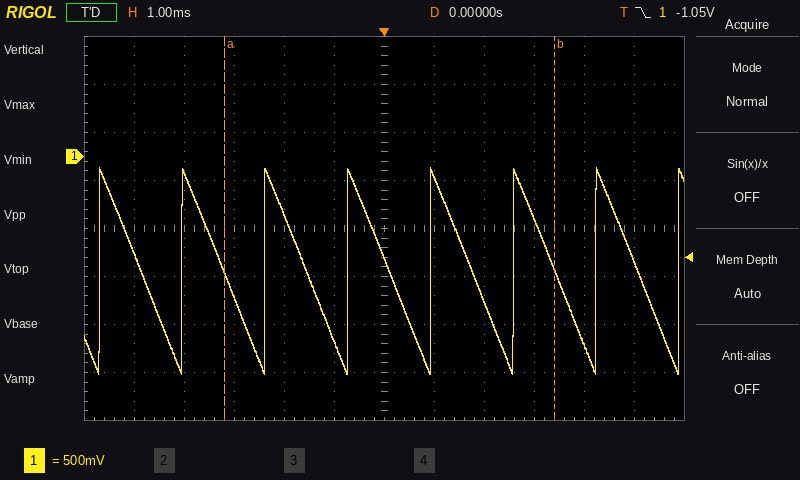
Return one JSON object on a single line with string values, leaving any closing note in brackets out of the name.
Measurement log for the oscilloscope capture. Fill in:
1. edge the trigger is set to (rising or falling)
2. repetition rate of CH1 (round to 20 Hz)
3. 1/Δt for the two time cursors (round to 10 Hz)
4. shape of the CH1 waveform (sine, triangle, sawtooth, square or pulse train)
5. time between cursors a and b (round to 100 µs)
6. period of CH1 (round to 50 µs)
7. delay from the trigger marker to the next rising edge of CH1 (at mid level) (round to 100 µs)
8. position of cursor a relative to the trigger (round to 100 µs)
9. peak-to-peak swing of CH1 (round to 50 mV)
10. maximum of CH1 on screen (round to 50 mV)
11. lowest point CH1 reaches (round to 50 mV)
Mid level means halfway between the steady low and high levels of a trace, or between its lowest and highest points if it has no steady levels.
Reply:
{"edge the trigger is set to": "falling", "repetition rate of CH1": "600 Hz", "1/Δt for the two time cursors": "150 Hz", "shape of the CH1 waveform": "sawtooth", "time between cursors a and b": "6.6 ms", "period of CH1": "1.65 ms", "delay from the trigger marker to the next rising edge of CH1 (at mid level)": "900 µs", "position of cursor a relative to the trigger": "-3.2 ms", "peak-to-peak swing of CH1": "2.15 V", "maximum of CH1 on screen": "-100 mV", "lowest point CH1 reaches": "-2.25 V"}
